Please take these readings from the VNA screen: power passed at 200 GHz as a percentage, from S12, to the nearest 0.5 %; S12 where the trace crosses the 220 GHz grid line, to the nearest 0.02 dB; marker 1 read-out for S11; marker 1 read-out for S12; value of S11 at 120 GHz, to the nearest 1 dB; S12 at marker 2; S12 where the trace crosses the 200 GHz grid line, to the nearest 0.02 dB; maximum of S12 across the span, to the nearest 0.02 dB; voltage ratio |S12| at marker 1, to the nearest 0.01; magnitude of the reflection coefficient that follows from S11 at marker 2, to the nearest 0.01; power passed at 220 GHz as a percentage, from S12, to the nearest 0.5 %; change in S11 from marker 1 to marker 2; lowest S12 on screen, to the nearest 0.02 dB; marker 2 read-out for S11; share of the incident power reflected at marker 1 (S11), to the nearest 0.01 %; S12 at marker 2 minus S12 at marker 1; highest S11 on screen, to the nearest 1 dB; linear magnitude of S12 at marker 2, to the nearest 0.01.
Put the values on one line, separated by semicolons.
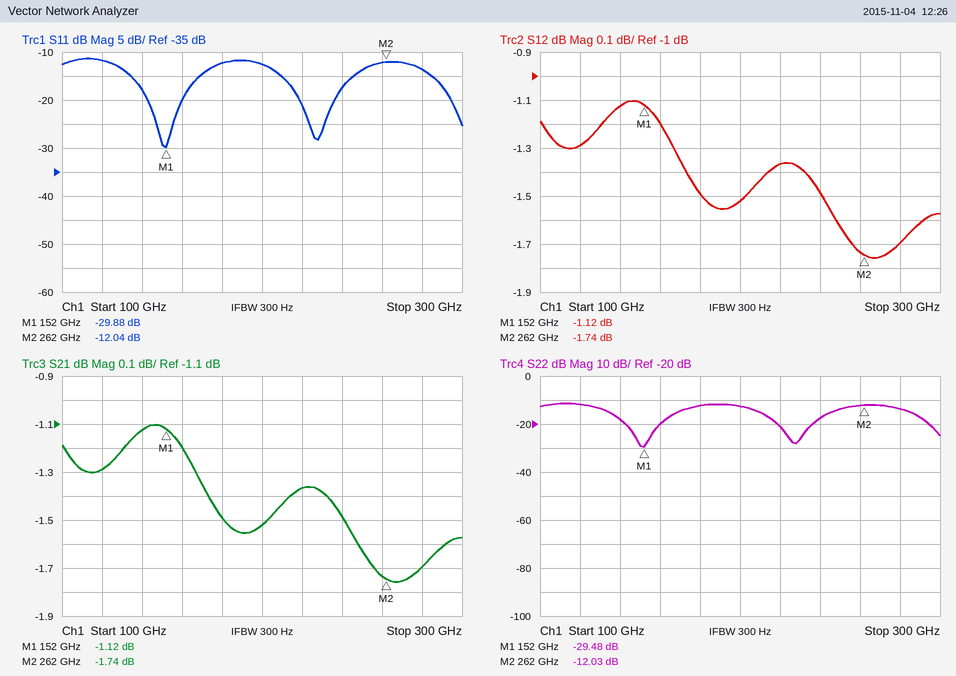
70.5 %; -1.36 dB; -29.88 dB; -1.12 dB; -12 dB; -1.74 dB; -1.52 dB; -1.10 dB; 0.88; 0.25; 73.0 %; 17.84 dB; -1.76 dB; -12.04 dB; 0.10 %; -0.62 dB; -11 dB; 0.82
